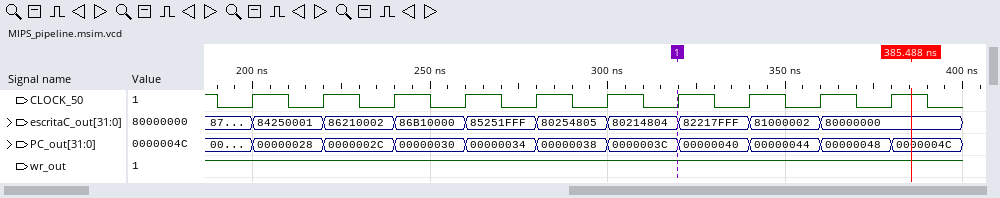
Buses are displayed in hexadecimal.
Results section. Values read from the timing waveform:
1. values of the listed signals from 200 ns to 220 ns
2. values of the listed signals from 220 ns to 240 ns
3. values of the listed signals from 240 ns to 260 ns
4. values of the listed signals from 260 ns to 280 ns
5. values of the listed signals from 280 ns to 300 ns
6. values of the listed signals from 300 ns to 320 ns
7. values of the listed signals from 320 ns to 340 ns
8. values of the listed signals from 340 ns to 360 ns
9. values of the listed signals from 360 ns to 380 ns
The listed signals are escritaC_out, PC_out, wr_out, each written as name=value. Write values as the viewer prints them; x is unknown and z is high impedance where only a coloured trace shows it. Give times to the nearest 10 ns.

escritaC_out=84250001, PC_out=00000028, wr_out=1
escritaC_out=86210002, PC_out=0000002C, wr_out=1
escritaC_out=86B10000, PC_out=00000030, wr_out=1
escritaC_out=85251FFF, PC_out=00000034, wr_out=1
escritaC_out=80254805, PC_out=00000038, wr_out=1
escritaC_out=80214804, PC_out=0000003C, wr_out=1
escritaC_out=82217FFF, PC_out=00000040, wr_out=1
escritaC_out=81000002, PC_out=00000044, wr_out=1
escritaC_out=80000000, PC_out=00000048, wr_out=1
